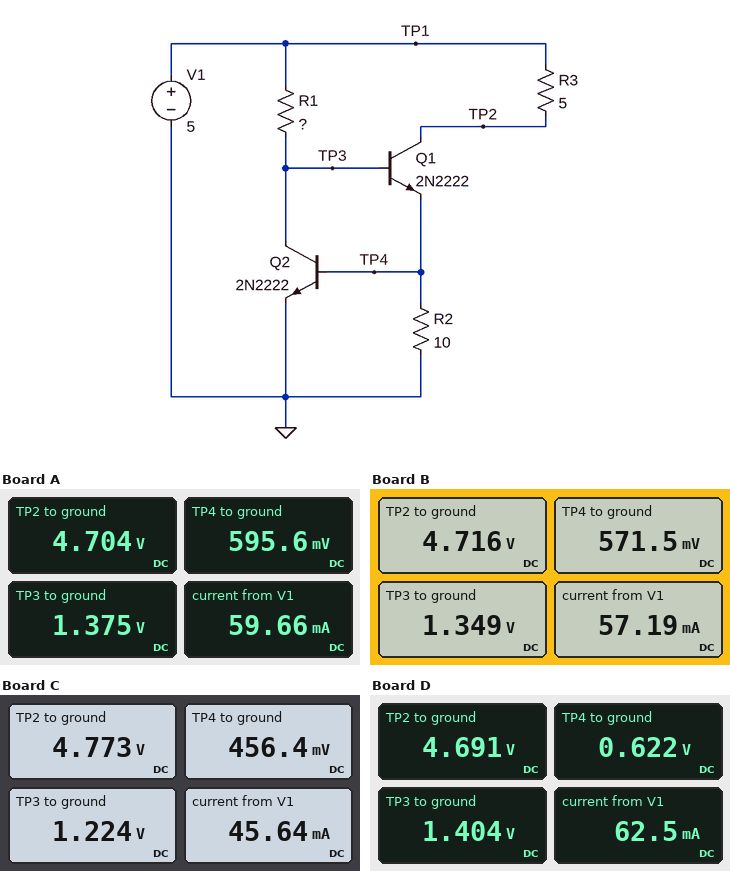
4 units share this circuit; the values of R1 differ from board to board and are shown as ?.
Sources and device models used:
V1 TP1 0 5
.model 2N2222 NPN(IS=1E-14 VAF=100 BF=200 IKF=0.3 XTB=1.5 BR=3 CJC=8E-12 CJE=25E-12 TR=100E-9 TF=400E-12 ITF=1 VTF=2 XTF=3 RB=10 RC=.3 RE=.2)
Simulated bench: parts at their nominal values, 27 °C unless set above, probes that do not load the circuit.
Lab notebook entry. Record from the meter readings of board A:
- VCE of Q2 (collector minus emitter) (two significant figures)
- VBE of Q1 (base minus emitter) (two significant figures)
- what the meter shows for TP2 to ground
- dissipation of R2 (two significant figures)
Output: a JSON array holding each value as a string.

["1.4 V", "780 mV", "4.704 V", "35 mW"]
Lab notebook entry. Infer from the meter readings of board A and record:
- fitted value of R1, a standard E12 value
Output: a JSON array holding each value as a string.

["8.2 kΩ"]
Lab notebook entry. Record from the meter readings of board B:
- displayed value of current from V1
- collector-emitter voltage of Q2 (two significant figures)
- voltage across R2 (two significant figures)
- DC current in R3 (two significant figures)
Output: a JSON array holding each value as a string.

["57.19 mA", "1.3 V", "570 mV", "57 mA"]
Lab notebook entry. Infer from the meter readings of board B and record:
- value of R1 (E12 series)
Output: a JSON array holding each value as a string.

["10 kΩ"]
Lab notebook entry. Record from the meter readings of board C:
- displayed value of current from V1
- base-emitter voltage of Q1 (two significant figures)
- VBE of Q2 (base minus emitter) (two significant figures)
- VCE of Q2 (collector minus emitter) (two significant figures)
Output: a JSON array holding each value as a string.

["45.64 mA", "770 mV", "460 mV", "1.2 V"]
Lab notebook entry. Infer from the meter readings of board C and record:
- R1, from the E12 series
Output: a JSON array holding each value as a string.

["15 kΩ"]
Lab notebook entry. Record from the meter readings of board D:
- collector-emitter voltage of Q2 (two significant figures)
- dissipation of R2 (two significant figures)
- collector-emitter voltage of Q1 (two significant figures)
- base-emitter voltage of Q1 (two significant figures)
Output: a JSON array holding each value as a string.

["1.4 V", "39 mW", "4.1 V", "780 mV"]
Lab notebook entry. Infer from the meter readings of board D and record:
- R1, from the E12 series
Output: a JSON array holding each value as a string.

["5.6 kΩ"]
